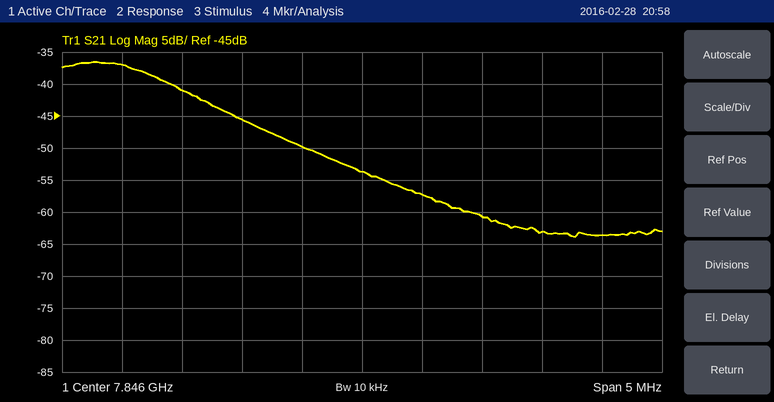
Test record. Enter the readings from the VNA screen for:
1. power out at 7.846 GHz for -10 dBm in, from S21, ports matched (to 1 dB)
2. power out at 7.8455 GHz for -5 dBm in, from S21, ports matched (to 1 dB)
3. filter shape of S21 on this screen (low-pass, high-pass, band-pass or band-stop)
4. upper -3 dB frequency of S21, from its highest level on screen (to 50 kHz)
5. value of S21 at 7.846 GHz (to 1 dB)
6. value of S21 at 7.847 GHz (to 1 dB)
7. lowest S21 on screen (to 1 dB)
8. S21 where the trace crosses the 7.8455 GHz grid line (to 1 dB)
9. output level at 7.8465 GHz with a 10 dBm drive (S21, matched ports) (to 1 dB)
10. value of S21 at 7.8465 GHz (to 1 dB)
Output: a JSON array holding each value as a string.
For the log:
["-64 dBm", "-55 dBm", "low-pass", "7.84435 GHz", "-54 dB", "-61 dB", "-64 dB", "-50 dB", "-47 dBm", "-57 dB"]
